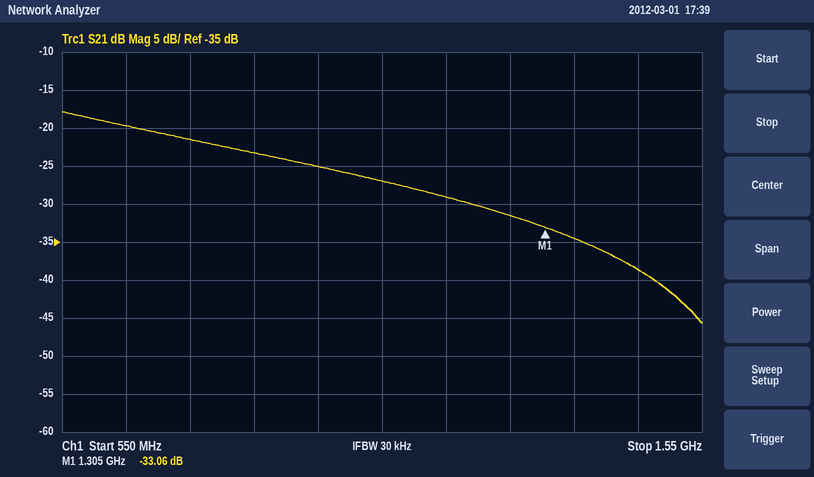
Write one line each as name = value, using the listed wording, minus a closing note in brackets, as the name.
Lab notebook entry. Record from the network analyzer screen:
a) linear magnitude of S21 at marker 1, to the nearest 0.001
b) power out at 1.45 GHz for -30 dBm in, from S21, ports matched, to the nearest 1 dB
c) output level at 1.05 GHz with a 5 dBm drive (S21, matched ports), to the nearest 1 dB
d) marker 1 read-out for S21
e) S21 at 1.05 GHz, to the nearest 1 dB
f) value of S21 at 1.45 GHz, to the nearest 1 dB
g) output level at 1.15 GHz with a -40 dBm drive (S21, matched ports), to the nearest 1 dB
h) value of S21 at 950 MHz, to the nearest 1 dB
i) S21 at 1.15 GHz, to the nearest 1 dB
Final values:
linear magnitude of S21 at marker 1, to the nearest 0.001 = 0.022
power out at 1.45 GHz for -30 dBm in, from S21, ports matched, to the nearest 1 dB = -69 dBm
output level at 1.05 GHz with a 5 dBm drive (S21, matched ports), to the nearest 1 dB = -22 dBm
marker 1 read-out for S21 = -33.06 dB
S21 at 1.05 GHz, to the nearest 1 dB = -27 dB
value of S21 at 1.45 GHz, to the nearest 1 dB = -39 dB
output level at 1.15 GHz with a -40 dBm drive (S21, matched ports), to the nearest 1 dB = -69 dBm
value of S21 at 950 MHz, to the nearest 1 dB = -25 dB
S21 at 1.15 GHz, to the nearest 1 dB = -29 dB
